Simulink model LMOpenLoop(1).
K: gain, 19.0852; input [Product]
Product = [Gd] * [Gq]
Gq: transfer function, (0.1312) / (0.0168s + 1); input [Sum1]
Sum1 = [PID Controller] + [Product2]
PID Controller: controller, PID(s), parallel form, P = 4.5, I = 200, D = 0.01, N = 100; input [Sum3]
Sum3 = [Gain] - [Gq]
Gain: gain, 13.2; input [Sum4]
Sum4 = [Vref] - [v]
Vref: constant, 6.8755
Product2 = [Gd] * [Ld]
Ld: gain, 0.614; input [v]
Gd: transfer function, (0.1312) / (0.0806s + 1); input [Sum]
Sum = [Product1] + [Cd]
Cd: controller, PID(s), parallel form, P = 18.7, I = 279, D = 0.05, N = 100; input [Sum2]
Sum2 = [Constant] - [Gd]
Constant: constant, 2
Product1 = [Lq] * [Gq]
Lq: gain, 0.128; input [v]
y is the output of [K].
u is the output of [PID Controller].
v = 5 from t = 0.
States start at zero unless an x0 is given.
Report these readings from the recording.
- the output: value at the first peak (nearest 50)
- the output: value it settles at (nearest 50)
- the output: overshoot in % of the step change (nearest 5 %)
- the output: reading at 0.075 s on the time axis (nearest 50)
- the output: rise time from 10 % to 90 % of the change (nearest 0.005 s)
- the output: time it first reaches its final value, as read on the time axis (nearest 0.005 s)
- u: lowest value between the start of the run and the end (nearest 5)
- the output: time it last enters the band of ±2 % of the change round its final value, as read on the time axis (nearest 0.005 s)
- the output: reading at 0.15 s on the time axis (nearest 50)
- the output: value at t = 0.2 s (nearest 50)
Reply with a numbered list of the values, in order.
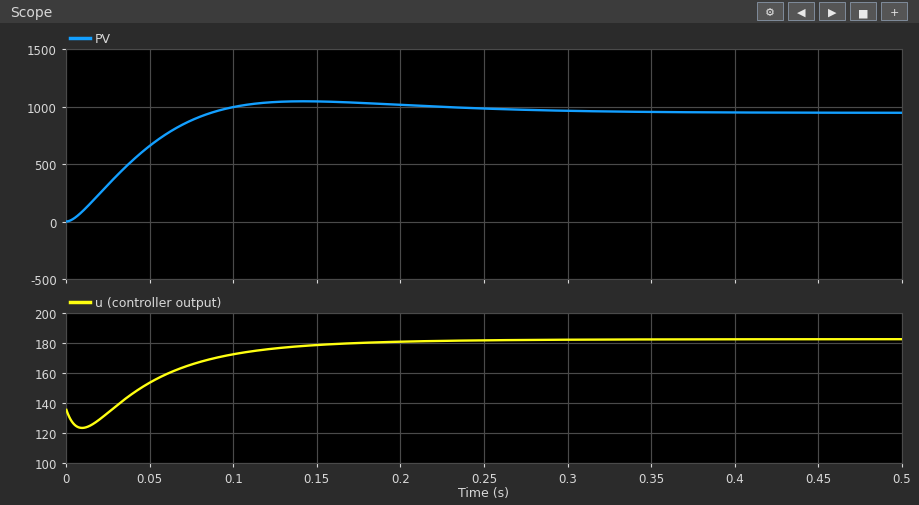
1. 1050
2. 950
3. 10 %
4. 900
5. 0.060 s
6. 0.085 s
7. 125
8. 0.295 s
9. 1050
10. 1000
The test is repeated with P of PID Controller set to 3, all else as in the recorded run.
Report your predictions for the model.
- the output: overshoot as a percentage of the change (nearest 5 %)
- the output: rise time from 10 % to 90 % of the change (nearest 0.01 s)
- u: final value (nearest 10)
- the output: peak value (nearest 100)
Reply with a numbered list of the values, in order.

1. 15 %
2. 0.06 s
3. 180
4. 1100
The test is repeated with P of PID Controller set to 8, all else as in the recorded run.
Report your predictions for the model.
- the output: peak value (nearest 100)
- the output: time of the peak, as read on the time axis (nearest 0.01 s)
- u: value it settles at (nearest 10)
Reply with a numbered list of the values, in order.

1. 1000
2. 0.15 s
3. 180
